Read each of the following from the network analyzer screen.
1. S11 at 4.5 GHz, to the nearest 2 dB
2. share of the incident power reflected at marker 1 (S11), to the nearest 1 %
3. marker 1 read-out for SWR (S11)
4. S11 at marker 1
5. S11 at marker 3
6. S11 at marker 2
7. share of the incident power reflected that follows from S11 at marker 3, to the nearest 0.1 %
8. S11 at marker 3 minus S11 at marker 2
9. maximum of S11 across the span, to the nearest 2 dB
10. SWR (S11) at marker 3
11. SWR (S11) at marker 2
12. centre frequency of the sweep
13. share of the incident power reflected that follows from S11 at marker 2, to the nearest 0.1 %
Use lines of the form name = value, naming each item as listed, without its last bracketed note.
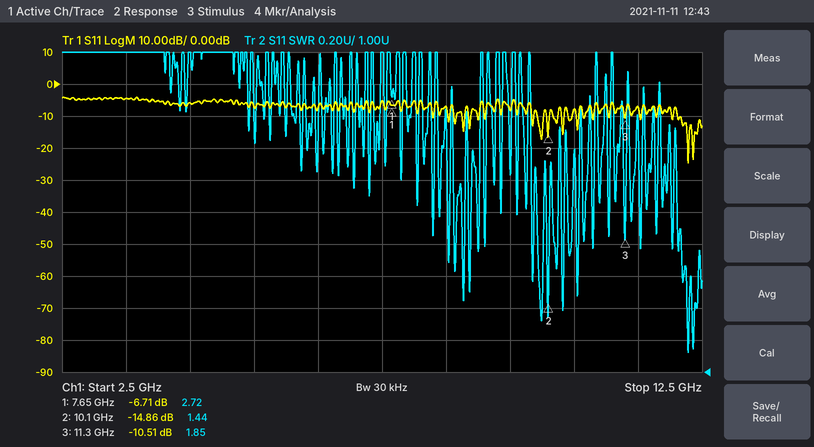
S11 at 4.5 GHz, to the nearest 2 dB = -6 dB
share of the incident power reflected at marker 1 (S11), to the nearest 1 % = 21 %
marker 1 read-out for SWR = 2.72
S11 at marker 1 = -6.71 dB
S11 at marker 3 = -10.51 dB
S11 at marker 2 = -14.86 dB
share of the incident power reflected that follows from S11 at marker 3, to the nearest 0.1 % = 8.9 %
S11 at marker 3 minus S11 at marker 2 = 4.35 dB
maximum of S11 across the span, to the nearest 2 dB = -4 dB
SWR (S11) at marker 3 = 1.85
SWR (S11) at marker 2 = 1.44
centre frequency of the sweep = 7.5 GHz
share of the incident power reflected that follows from S11 at marker 2, to the nearest 0.1 % = 3.3 %
